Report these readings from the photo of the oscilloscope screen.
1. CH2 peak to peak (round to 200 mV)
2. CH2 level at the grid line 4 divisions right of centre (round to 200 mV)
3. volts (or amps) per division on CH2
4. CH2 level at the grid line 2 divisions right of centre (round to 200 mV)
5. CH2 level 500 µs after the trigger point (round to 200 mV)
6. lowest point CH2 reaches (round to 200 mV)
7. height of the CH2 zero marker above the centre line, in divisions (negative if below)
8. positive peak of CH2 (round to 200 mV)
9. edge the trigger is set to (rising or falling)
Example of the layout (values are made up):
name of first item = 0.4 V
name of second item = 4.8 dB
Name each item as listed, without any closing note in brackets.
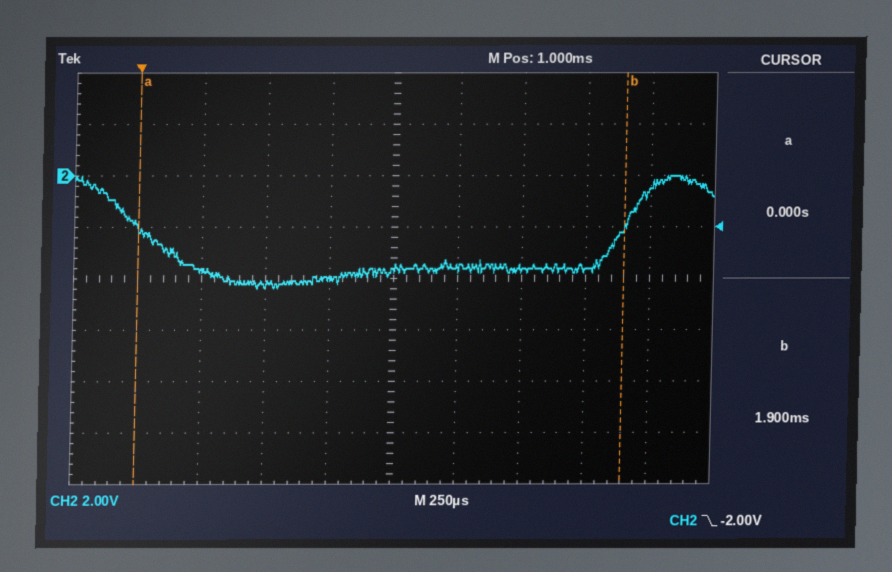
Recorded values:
CH2 peak to peak = 4.4 V
CH2 level at the grid line 4 divisions right of centre = -400 mV
volts (or amps) per division on CH2 = 2 V
CH2 level at the grid line 2 divisions right of centre = -3.6 V
CH2 level 500 µs after the trigger point = -4.2 V
lowest point CH2 reaches = -4.4 V
height of the CH2 zero marker above the centre line, in divisions = +2.0 div
positive peak of CH2 = 0.0 V
edge the trigger is set to = falling
